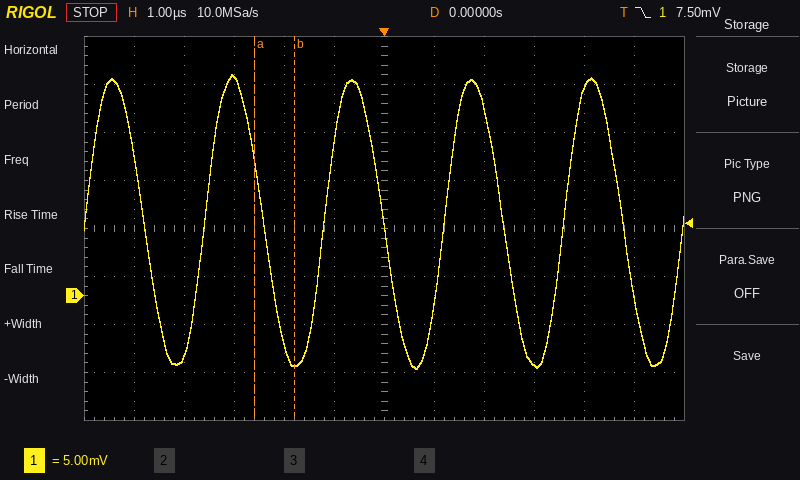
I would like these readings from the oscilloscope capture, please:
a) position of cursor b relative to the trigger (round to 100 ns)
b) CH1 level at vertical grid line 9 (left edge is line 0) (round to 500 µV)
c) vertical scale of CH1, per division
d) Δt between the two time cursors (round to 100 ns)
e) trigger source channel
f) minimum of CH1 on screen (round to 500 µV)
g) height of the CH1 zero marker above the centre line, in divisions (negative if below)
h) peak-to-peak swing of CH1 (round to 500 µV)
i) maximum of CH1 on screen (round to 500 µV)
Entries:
-1.8 µs
-7.0 mV
5 mV
800 ns
CH1
-7.5 mV
-1.4 div
30.5 mV
23.0 mV
